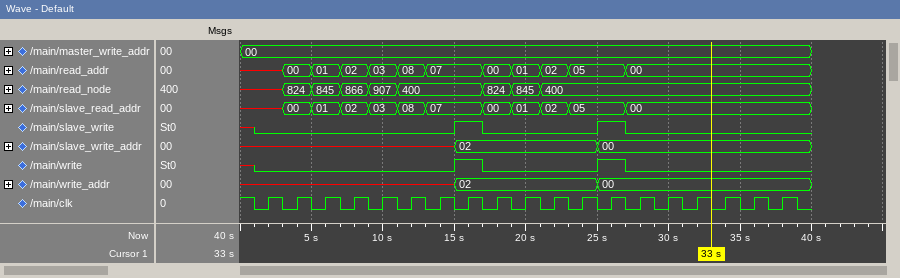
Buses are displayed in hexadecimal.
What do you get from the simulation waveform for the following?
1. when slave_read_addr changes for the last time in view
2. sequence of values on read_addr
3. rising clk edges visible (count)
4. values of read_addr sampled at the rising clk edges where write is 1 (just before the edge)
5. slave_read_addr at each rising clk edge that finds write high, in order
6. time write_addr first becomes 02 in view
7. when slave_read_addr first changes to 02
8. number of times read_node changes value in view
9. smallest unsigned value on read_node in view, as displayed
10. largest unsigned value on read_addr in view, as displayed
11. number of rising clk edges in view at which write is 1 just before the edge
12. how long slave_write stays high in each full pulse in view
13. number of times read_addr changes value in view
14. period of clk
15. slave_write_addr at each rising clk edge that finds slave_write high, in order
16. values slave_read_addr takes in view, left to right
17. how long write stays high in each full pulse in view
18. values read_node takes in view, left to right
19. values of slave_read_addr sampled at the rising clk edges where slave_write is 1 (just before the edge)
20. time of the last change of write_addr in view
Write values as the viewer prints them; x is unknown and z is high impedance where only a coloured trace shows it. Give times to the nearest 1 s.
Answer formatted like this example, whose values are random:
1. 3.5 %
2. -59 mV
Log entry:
1. 27 s
2. x, 00, 01, 02, 03, 08, 07, 00, 01, 02, 05, 00
3. 19
4. 07, 05
5. 07, 05
6. 15 s
7. 7 s
8. 8
9. 400
10. 08
11. 2
12. 2 s, 2 s
13. 11
14. 2 s
15. 02, 00
16. x, 00, 01, 02, 03, 08, 07, 00, 01, 02, 05, 00
17. 2 s, 2 s
18. x, 824, 845, 866, 907, 400, 824, 845, 400
19. 07, 05
20. 25 s
